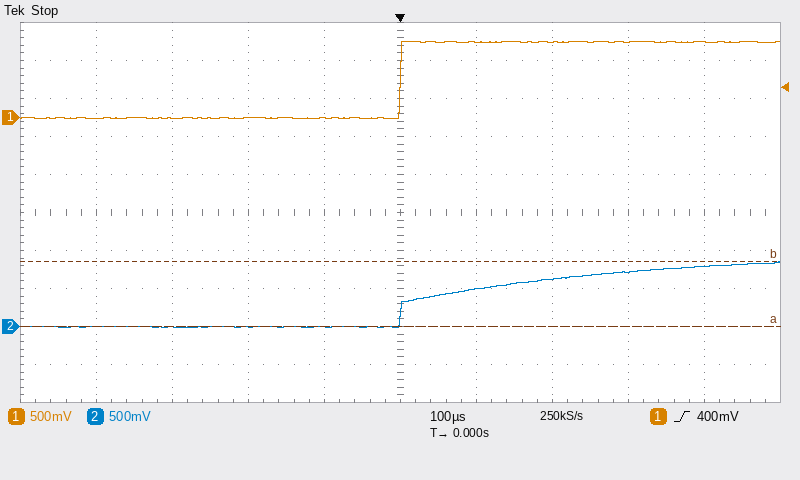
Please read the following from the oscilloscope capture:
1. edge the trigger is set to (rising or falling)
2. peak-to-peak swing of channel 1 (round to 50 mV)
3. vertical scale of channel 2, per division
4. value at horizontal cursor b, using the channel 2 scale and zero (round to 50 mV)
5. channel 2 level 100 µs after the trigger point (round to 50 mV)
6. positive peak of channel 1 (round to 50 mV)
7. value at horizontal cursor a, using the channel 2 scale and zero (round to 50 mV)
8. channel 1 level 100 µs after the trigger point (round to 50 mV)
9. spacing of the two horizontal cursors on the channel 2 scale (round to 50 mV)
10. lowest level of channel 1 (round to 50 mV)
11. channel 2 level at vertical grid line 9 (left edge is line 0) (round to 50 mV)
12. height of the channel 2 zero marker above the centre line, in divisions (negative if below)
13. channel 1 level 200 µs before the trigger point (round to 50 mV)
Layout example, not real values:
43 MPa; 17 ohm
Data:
rising; 1.00 V; 500 mV; 850 mV; 500 mV; 1.00 V; 0 mV; 1.00 V; 850 mV; 0 mV; 800 mV; -3.0 div; 0 mV
